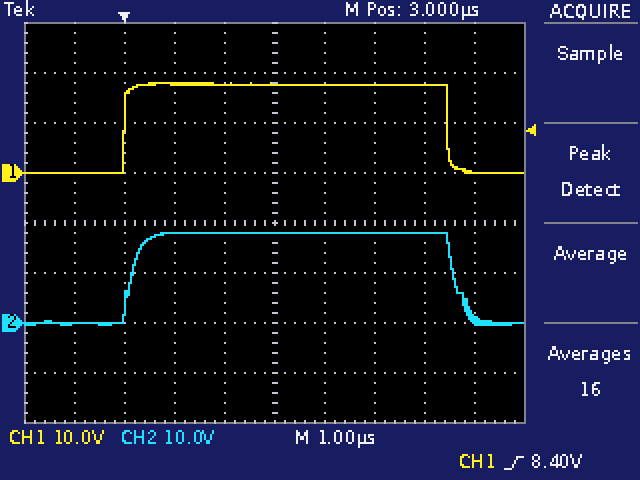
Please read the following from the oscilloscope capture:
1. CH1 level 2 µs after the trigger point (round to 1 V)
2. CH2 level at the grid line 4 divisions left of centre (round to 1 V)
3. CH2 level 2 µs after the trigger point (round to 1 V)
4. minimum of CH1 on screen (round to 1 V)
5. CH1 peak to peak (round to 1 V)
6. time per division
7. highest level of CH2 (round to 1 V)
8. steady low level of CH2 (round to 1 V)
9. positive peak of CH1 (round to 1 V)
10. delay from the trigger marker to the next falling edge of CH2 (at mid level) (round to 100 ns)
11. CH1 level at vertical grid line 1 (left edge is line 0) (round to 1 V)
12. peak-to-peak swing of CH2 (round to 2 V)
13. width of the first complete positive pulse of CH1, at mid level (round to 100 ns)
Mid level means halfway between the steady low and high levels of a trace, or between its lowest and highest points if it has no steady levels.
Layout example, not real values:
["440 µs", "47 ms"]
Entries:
["18 V", "0 V", "18 V", "0 V", "18 V", "1 µs", "18 V", "0 V", "18 V", "6.6 µs", "0 V", "18 V", "6.5 µs"]
